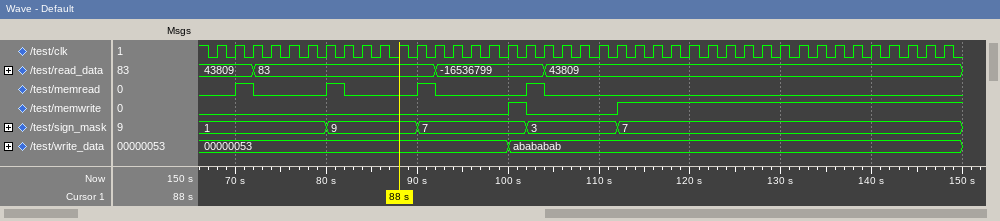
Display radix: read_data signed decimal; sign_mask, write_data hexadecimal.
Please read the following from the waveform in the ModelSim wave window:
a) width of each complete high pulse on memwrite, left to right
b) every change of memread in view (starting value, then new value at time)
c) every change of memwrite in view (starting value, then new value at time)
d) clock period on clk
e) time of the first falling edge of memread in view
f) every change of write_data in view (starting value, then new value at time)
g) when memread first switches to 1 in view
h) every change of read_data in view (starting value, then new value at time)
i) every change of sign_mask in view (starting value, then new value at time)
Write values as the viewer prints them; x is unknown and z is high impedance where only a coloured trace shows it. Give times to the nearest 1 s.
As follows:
2 s
0, 1 at 70 s, 0 at 72 s, 1 at 80 s, 0 at 82 s, 1 at 90 s, 0 at 92 s, 1 at 102 s, 0 at 104 s
0, 1 at 100 s, 0 at 102 s, 1 at 112 s
2 s
72 s
00000053, abababab at 100 s
70 s
43809, 83 at 72 s, -16536799 at 92 s, 43809 at 104 s
1, 9 at 80 s, 7 at 90 s, 3 at 102 s, 7 at 112 s
